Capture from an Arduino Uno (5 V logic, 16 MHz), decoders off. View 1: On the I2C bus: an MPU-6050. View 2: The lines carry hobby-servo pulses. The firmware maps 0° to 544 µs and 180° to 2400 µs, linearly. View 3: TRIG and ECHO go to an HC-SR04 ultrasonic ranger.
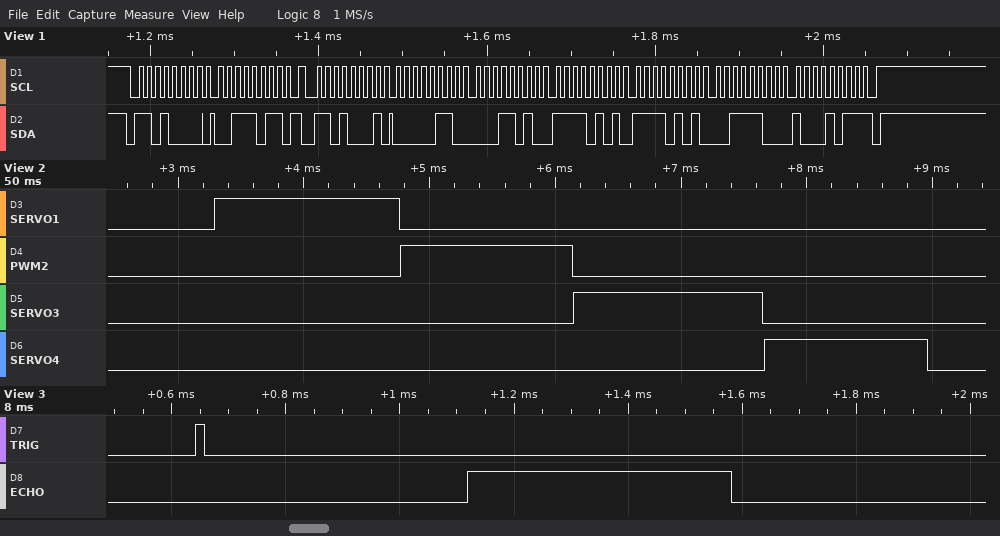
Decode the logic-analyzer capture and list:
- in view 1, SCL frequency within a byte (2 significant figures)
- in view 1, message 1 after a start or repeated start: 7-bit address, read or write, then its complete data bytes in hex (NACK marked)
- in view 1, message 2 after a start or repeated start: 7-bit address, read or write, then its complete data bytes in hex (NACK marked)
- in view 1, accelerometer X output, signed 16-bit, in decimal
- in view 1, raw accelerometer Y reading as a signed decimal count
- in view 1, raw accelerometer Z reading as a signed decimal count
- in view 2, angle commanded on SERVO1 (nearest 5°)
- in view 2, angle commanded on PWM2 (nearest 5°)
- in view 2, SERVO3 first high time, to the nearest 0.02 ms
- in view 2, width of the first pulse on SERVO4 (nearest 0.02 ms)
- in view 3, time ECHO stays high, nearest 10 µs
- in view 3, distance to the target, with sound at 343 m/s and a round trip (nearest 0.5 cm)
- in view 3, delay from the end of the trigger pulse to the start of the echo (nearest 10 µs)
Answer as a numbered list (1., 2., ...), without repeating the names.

1. 100 kHz
2. 0x68 write: 3B
3. 0x68 read: 06 1A F5 F5 3C 8B NACK
4. 1562
5. -2571
6. 15499
7. 90°
8. 80°
9. 1.50 ms
10. 1.30 ms
11. 460 µs
12. 8 cm
13. 460 µs
